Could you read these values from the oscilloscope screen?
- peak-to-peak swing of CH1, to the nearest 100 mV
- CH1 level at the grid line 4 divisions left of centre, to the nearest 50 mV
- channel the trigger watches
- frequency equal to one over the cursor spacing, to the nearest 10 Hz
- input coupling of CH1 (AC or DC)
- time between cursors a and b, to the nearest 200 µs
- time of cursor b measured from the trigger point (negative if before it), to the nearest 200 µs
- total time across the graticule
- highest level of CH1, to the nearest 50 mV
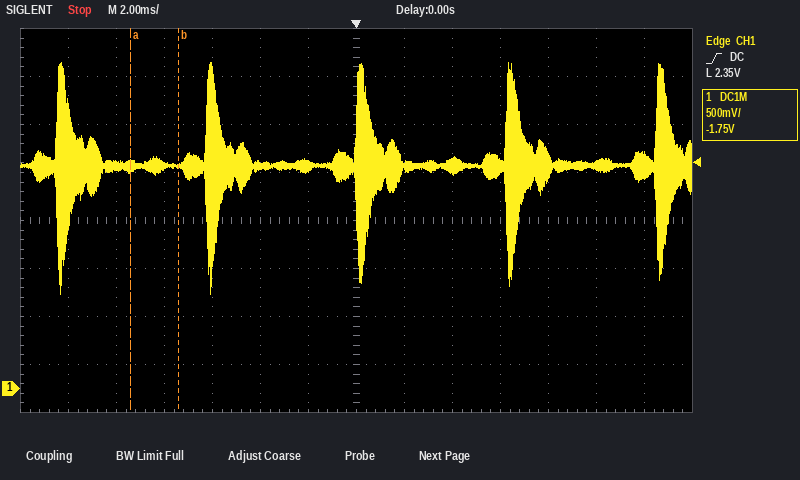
2.40 V
2.30 V
CH1
500 Hz
DC
2.0 ms
-7.4 ms
28 ms
3.40 V
